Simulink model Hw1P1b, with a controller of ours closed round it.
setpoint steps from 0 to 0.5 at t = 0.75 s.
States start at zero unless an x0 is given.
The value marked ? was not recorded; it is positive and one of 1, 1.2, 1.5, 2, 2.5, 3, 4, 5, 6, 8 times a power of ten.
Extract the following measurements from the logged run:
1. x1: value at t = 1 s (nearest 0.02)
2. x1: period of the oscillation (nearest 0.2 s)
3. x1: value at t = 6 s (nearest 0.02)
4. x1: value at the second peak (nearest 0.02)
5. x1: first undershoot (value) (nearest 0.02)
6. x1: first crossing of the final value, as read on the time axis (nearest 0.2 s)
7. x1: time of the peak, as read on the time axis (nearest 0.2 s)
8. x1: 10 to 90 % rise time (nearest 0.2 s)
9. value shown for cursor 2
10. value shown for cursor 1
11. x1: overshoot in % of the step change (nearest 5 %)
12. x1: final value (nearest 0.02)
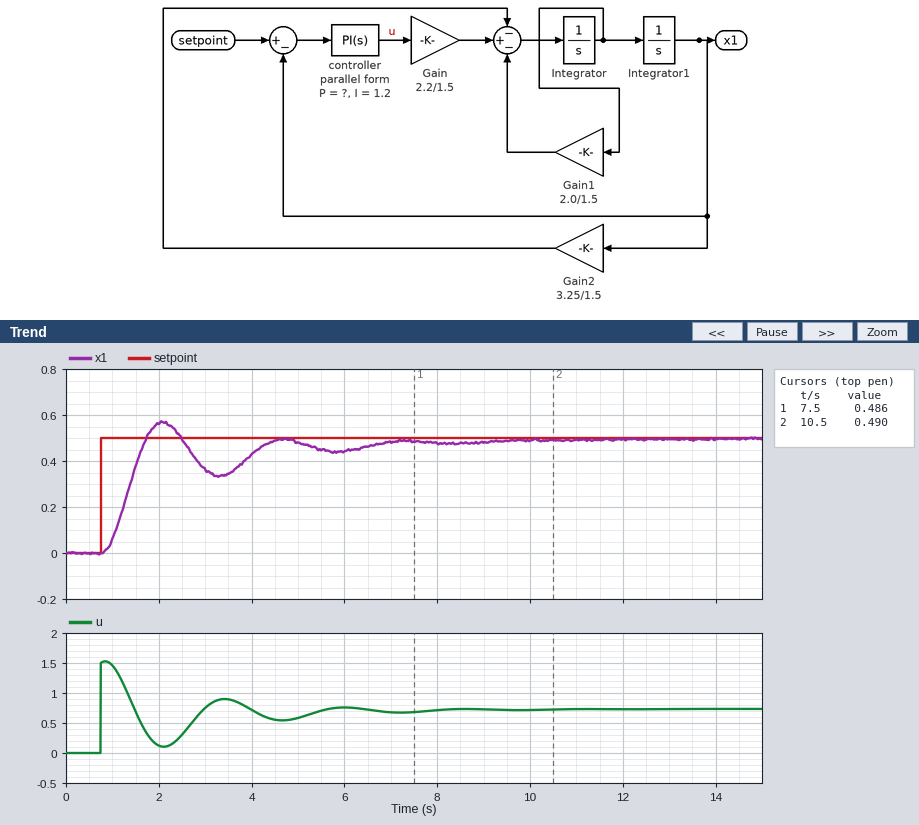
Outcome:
0.06
2.6 s
0.44
0.50
0.34
1.8 s
2.0 s
0.6 s
0.490
0.486
15 %
0.50
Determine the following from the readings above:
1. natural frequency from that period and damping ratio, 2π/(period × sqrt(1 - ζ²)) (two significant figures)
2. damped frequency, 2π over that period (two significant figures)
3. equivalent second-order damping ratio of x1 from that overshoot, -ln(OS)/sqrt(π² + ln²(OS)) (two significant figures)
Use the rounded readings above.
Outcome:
2.8 rad/s
2.4 rad/s
0.52
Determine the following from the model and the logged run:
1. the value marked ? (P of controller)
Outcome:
3
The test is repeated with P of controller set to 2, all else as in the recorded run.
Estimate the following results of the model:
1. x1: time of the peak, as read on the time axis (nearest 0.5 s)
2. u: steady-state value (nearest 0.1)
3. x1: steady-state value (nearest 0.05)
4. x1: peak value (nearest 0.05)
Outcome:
2.5 s
0.7
0.50
0.55
